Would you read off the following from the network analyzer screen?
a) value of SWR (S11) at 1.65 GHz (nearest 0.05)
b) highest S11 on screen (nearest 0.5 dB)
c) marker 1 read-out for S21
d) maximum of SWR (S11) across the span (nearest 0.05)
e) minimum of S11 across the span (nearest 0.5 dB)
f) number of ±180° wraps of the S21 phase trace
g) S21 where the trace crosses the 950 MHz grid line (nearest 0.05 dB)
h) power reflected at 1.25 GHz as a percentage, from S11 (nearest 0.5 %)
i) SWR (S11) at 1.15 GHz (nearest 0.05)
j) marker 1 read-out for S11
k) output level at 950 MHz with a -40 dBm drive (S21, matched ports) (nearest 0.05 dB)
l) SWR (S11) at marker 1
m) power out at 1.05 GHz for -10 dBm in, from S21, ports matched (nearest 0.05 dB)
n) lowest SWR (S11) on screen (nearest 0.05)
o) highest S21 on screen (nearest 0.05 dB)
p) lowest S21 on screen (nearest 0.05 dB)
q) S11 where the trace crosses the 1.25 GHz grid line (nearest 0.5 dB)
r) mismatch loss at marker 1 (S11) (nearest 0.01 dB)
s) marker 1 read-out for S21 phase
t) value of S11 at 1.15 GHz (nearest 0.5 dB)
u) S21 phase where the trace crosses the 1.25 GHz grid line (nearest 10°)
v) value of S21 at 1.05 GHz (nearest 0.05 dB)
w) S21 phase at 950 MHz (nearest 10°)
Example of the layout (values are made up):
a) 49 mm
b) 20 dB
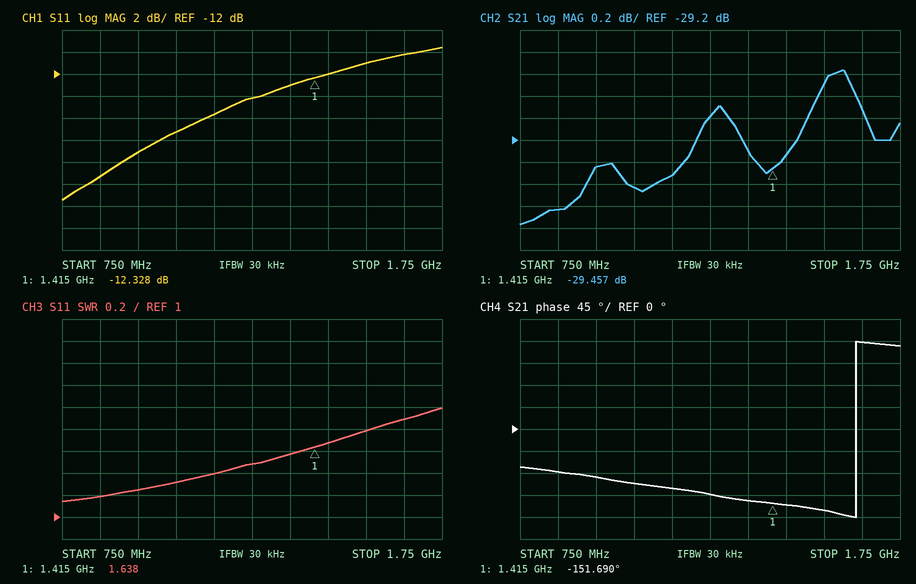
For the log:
a) 1.90
b) -9.5 dB
c) -29.457 dB
d) 2.00
e) -23.5 dB
f) 1
g) -29.45 dB
h) 4.0 %
i) 1.40
j) -12.328 dB
k) -69.45 dBm
l) 1.638
m) -39.65 dBm
n) 1.15
o) -28.55 dB
p) -29.95 dB
q) -14.0 dB
r) 0.26 dB
s) -151.690°
t) -15.5 dB
u) -130°
v) -29.65 dB
w) -100°
